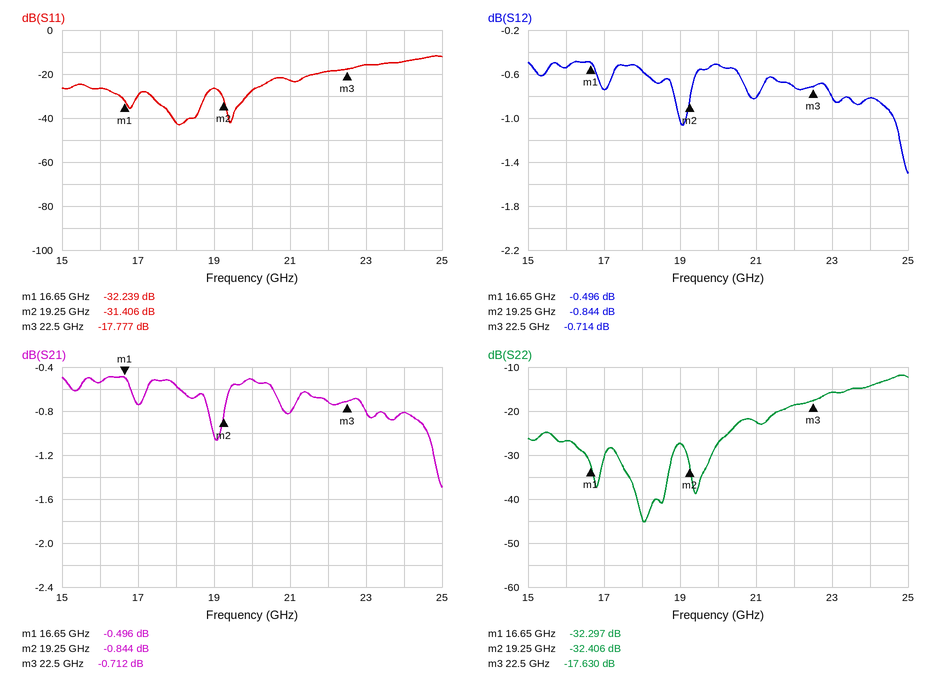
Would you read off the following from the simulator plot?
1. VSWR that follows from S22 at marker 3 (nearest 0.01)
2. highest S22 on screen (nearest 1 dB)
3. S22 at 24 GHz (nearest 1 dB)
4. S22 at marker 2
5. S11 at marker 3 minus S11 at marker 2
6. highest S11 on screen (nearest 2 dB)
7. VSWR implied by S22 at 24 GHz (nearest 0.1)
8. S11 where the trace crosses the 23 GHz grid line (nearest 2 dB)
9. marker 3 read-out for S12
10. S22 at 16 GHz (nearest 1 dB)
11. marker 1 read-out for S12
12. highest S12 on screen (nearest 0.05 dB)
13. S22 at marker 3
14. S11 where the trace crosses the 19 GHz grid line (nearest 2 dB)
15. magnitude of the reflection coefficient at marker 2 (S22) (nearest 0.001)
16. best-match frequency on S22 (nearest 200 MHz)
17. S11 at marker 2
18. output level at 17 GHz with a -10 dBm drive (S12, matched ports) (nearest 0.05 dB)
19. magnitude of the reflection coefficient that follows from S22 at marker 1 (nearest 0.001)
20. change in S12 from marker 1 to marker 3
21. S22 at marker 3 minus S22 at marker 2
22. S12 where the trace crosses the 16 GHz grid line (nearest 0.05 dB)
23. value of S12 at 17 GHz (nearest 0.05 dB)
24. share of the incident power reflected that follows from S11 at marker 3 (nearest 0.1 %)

1.30
-12 dB
-14 dB
-32.406 dB
13.629 dB
-12 dB
1.5
-16 dB
-0.714 dB
-27 dB
-0.496 dB
-0.50 dB
-17.630 dB
-26 dB
0.024
18.0 GHz
-31.406 dB
-10.75 dBm
0.024
-0.218 dB
14.776 dB
-0.55 dB
-0.75 dB
1.7 %
